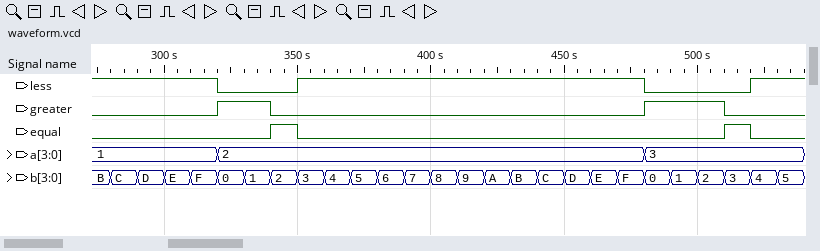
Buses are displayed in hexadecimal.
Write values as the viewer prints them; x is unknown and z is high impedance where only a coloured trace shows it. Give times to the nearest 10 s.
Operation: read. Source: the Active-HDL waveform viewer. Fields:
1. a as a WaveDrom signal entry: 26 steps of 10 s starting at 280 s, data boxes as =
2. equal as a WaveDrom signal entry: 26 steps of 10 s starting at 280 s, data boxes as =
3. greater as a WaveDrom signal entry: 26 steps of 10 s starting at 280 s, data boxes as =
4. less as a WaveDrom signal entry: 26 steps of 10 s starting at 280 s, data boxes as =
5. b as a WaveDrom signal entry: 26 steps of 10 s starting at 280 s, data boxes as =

{name: 'a', wave: '=...=...............=.....', data: '1 2 3'}
{name: 'equal', wave: '0.....10...............10.'}
{name: 'greater', wave: '0...1.0.............1..0..'}
{name: 'less', wave: '1...0..1............0...1.'}
{name: 'b', wave: '==========================', data: 'C D E F 0 1 2 3 4 5 6 7 8 9 A B C D E F 0 1 2 3 4 5'}
